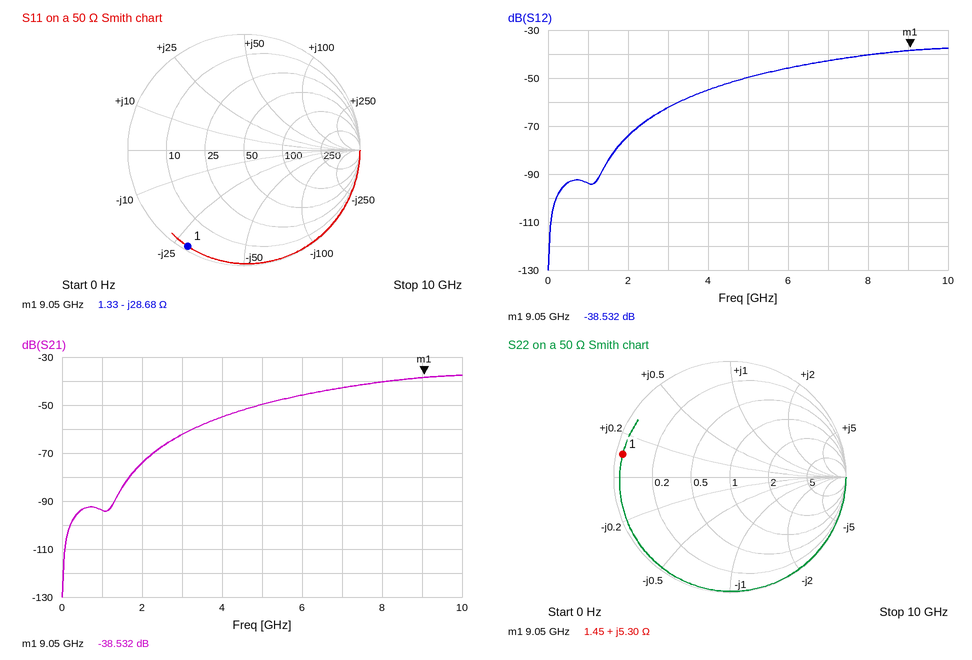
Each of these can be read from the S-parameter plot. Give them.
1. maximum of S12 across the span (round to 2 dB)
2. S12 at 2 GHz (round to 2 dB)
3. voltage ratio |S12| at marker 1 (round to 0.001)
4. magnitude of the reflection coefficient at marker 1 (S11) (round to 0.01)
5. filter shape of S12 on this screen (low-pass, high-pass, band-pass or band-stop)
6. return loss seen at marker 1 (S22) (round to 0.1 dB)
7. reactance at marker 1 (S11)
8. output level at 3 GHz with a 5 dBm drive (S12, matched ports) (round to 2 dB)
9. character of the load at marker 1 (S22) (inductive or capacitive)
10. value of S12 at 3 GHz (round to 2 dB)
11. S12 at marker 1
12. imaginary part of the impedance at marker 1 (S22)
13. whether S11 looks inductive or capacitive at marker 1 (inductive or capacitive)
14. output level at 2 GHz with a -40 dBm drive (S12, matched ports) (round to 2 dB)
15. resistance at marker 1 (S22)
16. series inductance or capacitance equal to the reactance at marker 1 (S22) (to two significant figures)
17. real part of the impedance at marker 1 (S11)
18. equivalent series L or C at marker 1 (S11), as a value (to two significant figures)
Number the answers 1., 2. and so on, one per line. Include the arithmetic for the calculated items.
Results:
1. -38 dB
2. -74 dB
3. 10^(-38.532/20) ≈ 0.012
4. 0.96
5. high-pass
6. 0.5 dB
7. -28.68 Ω
8. 5 dBm + (-62 dB) = -58 dBm
9. inductive
10. -62 dB
11. -38.532 dB
12. +5.30 Ω
13. capacitive
14. -40 dBm + (-74 dB) = -114 dBm
15. 1.45 Ω
16. L = 5.3 Ω/(2π × 9.05 GHz) ≈ 93 pH
17. 1.33 Ω
18. C = 1/(2π × 9.05 GHz × 28.68 Ω) ≈ 613 fF, so 610 fF to two significant figures
